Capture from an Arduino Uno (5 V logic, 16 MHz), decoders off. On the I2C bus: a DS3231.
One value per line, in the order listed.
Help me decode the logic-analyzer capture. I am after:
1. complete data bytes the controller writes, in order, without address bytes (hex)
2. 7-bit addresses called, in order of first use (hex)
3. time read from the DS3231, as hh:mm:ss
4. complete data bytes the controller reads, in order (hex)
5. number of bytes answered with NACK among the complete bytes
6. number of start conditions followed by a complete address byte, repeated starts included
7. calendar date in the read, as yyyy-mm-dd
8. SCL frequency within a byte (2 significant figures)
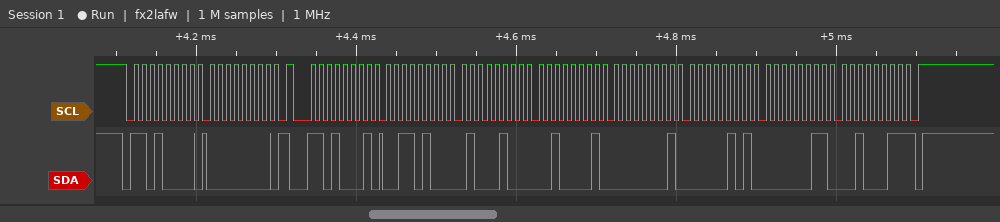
00
0x68
21:44:34
34 44 21 01 05 03 23
1
2
2023-03-05
100 kHz
